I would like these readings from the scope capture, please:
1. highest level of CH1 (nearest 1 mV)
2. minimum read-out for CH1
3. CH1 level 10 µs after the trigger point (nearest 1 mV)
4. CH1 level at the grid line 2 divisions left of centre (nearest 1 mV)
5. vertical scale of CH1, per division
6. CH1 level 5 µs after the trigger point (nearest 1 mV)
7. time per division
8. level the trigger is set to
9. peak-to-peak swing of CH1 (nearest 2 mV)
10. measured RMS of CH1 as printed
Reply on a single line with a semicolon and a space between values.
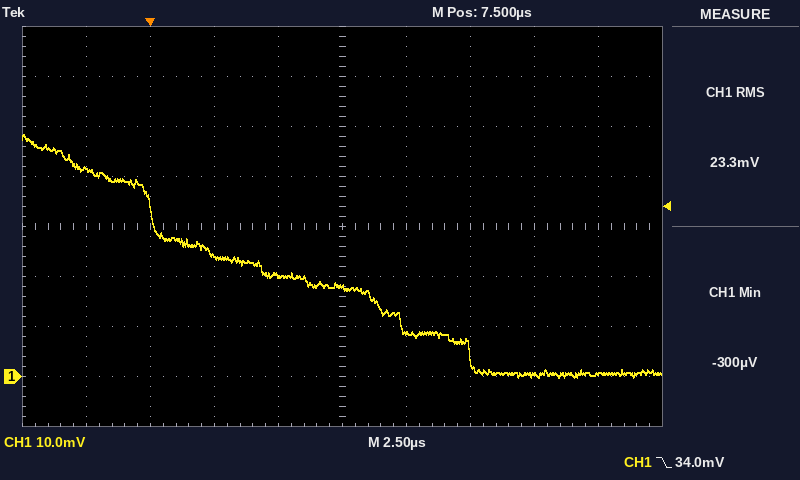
48 mV; -300 µV; 9 mV; 24 mV; 10 mV; 20 mV; 2.5 µs; 34.0 mV; 48 mV; 23.3 mV
